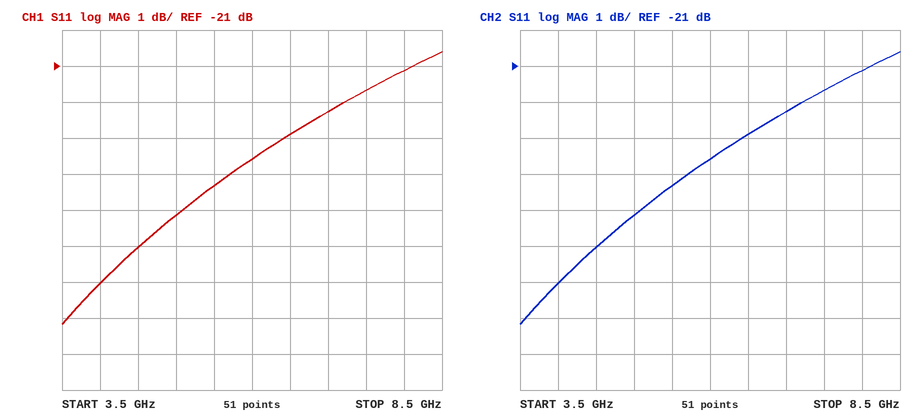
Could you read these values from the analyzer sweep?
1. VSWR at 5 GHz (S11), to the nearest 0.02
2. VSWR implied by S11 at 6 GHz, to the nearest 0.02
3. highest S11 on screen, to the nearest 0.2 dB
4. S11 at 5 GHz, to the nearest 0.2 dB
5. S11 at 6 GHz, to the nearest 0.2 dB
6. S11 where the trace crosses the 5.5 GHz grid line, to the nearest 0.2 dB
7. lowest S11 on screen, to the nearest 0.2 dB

1.12
1.14
-20.6 dB
-25.2 dB
-23.6 dB
-24.4 dB
-28.2 dB
